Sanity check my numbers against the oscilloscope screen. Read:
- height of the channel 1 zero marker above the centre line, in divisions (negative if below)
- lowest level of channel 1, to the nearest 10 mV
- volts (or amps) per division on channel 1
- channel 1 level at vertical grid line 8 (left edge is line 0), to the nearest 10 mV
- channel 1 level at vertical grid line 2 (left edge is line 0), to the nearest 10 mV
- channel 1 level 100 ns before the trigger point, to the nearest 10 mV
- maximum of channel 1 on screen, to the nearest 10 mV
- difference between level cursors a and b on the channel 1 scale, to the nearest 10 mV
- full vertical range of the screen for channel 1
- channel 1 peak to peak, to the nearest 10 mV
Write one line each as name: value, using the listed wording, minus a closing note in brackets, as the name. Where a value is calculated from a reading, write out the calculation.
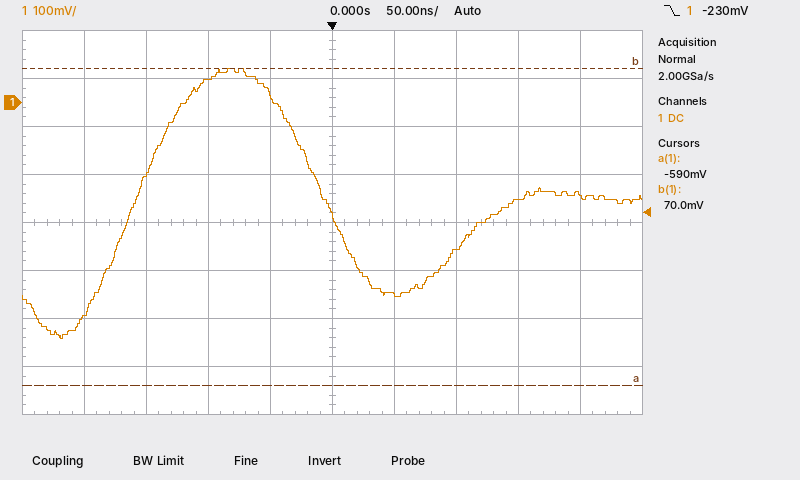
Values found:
height of the channel 1 zero marker above the centre line, in divisions: +2.5 div
lowest level of channel 1, to the nearest 10 mV: -490 mV
volts (or amps) per division on channel 1: 100 mV
channel 1 level at vertical grid line 8 (left edge is line 0), to the nearest 10 mV: -200 mV
channel 1 level at vertical grid line 2 (left edge is line 0), to the nearest 10 mV: -150 mV
channel 1 level 100 ns before the trigger point, to the nearest 10 mV: 50 mV
maximum of channel 1 on screen, to the nearest 10 mV: 70 mV
difference between level cursors a and b on the channel 1 scale, to the nearest 10 mV: 660 mV
full vertical range of the screen for channel 1: 800 mV
channel 1 peak to peak, to the nearest 10 mV: 70 mV − (-490 mV) = 560 mV
